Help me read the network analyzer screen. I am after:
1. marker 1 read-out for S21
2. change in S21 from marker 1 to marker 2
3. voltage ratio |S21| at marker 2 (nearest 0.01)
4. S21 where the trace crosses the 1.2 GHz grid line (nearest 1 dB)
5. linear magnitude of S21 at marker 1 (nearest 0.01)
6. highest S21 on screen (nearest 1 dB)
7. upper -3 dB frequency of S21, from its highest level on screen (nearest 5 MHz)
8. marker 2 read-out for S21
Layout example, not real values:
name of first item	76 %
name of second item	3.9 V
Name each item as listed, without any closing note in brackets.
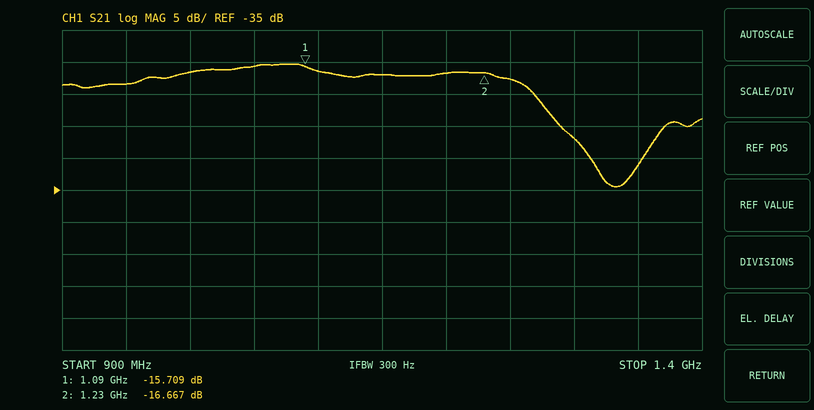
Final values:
marker 1 read-out for S21	-15.709 dB
change in S21 from marker 1 to marker 2	-0.958 dB
voltage ratio |S21| at marker 2	0.15
S21 where the trace crosses the 1.2 GHz grid line	-17 dB
linear magnitude of S21 at marker 1	0.16
highest S21 on screen	-15 dB
upper -3 dB frequency of S21, from its highest level on screen	1.260 GHz
marker 2 read-out for S21	-16.667 dB
